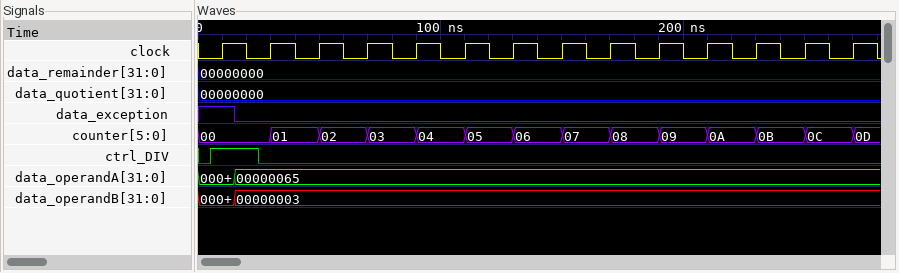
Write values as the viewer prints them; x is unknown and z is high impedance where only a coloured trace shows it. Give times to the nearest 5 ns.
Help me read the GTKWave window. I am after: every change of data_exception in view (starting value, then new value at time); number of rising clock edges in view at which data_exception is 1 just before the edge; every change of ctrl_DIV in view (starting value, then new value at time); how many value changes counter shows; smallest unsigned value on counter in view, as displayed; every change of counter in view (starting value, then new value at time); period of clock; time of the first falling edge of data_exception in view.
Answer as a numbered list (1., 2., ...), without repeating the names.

1. 1, 0 at 15 ns
2. 1
3. 0, 1 at 5 ns, 0 at 25 ns
4. 13
5. 00
6. 00, 01 at 30 ns, 02 at 50 ns, 03 at 70 ns, 04 at 90 ns, 05 at 110 ns, 06 at 130 ns, 07 at 150 ns, 08 at 170 ns, 09 at 190 ns, 0A at 210 ns, 0B at 230 ns, 0C at 250 ns, 0D at 270 ns
7. 20 ns
8. 15 ns
